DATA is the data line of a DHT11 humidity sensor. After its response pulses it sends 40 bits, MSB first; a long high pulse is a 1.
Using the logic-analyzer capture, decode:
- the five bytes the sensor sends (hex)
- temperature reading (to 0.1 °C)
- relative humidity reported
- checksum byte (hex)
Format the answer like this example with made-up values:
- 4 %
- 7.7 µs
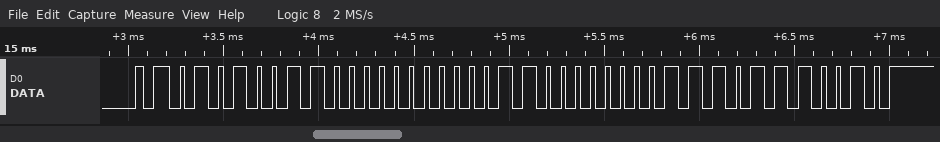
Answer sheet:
- 53 00 18 07 72
- 24.7 °C
- 83 %
- 0x72
